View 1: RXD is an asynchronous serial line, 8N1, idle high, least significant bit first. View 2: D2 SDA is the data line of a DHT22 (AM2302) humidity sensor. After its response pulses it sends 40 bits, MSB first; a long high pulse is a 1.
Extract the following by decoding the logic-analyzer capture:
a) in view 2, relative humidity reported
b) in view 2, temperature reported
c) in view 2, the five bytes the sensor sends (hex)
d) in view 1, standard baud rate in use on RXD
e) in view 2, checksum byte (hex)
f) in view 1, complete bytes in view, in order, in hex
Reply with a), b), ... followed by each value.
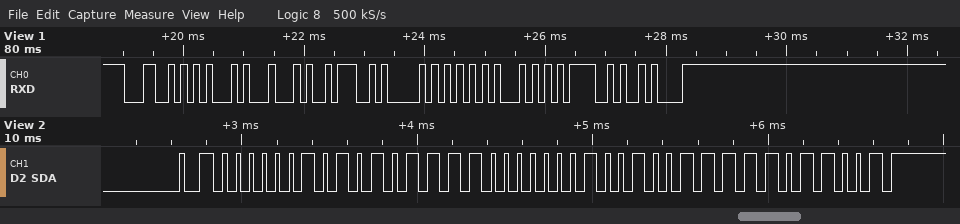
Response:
a) 68.7 %
b) 29.5 °C
c) 02 AF 01 27 D9
d) 9600 baud
e) 0xD9
f) 4C 45 44 3A 41 55 54 4F 0A
